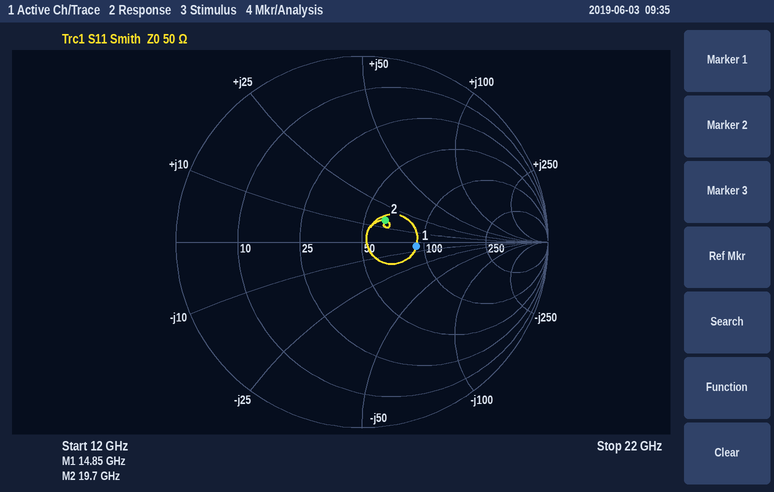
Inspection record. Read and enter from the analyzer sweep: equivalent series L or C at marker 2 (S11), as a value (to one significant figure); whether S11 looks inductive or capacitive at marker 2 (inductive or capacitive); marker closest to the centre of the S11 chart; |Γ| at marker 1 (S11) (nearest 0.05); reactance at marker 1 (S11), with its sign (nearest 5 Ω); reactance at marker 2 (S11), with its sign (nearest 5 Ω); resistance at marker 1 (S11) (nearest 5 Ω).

100 pH
inductive
marker 2
0.30
-5 Ω
+15 Ω
90 Ω
